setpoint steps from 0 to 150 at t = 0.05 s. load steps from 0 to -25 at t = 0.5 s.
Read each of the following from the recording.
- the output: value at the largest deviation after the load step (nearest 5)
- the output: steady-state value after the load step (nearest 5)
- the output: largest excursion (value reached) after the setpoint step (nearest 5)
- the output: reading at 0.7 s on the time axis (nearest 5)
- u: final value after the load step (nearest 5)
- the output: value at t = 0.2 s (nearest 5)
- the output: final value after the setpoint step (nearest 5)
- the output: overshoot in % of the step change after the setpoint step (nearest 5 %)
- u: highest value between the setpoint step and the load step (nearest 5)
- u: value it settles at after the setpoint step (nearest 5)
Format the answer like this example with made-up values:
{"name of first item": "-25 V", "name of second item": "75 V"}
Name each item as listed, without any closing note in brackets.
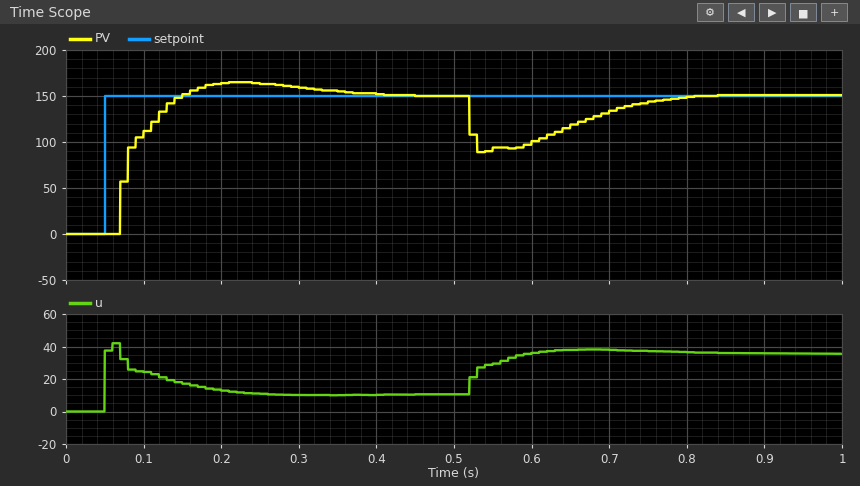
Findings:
{"the output: value at the largest deviation after the load step": "90", "the output: steady-state value after the load step": "150", "the output: largest excursion (value reached) after the setpoint step": "165", "the output: reading at 0.7 s on the time axis": "135", "u: final value after the load step": "35", "the output: value at t = 0.2 s": "165", "the output: final value after the setpoint step": "150", "the output: overshoot in % of the step change after the setpoint step": "10 %", "u: highest value between the setpoint step and the load step": "40", "u: value it settles at after the setpoint step": "10"}
